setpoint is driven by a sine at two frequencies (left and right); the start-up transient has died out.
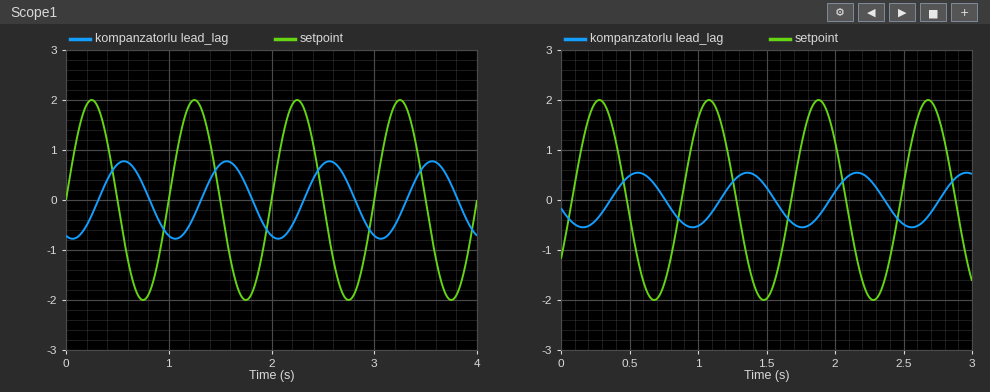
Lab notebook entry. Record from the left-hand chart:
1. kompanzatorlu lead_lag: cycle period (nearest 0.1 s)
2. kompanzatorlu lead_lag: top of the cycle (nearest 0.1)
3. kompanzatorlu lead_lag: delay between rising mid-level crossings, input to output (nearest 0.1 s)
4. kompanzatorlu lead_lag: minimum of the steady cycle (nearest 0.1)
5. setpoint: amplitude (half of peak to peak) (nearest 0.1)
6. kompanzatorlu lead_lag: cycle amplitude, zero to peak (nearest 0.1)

1.0 s
0.8
0.3 s
-0.8
2.0
0.8
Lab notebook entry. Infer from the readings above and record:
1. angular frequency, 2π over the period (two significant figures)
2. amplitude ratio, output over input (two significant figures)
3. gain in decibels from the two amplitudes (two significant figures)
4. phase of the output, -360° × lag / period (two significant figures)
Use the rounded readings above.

6.3 rad/s
0.40
-8.0 dB
-110°
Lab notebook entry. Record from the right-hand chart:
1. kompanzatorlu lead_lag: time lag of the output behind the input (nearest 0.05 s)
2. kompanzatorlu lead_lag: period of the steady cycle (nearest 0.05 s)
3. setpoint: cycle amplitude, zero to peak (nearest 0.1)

0.30 s
0.80 s
2.0
